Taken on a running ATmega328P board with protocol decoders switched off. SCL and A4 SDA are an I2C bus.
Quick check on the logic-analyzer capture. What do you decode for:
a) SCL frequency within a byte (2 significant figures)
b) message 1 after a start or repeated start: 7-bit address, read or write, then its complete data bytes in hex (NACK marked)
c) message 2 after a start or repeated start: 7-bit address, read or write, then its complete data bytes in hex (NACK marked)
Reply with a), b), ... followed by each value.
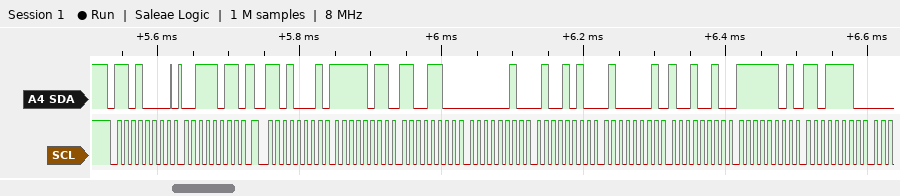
a) 100 kHz
b) 0x68 write: 3B
c) 0x68 read: FB CC 02 4A 41 92 FD DE
